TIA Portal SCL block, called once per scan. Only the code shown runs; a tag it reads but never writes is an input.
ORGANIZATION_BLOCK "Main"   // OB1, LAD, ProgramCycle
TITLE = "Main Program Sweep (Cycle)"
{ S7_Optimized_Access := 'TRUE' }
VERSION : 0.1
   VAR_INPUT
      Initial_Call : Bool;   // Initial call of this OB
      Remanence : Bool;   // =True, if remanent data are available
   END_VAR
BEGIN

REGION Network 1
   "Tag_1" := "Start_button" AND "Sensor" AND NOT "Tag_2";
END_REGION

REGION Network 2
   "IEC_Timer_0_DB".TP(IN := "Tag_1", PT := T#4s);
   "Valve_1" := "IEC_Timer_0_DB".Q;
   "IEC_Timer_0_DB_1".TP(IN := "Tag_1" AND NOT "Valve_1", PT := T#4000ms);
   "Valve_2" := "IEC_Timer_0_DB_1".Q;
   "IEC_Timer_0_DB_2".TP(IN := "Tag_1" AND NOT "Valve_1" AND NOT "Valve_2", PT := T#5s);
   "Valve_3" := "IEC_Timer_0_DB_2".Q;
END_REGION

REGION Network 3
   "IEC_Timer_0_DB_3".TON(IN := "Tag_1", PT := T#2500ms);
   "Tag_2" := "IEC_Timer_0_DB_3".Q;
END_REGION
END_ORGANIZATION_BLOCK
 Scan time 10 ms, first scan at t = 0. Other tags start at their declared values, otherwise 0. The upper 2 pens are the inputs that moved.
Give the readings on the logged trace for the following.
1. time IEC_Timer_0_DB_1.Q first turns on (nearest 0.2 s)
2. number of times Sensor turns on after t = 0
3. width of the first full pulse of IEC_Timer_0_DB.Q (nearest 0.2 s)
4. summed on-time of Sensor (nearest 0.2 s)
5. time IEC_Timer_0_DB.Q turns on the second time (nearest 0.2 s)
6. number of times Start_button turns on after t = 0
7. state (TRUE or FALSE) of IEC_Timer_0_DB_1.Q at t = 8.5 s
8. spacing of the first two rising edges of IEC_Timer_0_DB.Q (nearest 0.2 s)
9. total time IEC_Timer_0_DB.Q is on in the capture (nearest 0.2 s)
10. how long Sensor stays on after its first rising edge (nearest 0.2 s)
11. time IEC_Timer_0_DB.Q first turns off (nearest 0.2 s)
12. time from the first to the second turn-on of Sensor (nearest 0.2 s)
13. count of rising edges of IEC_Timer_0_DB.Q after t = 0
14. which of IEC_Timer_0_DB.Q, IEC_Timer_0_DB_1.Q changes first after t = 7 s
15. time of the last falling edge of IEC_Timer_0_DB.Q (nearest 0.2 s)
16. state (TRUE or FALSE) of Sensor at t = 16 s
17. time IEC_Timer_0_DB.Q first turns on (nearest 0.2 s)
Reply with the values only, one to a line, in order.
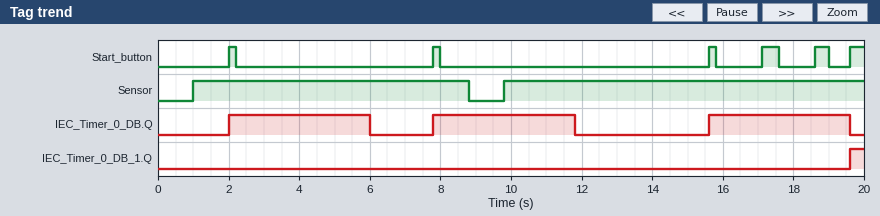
19.6 s
2
4.0 s
18.0 s
7.8 s
6
FALSE
5.8 s
12.0 s
7.8 s
6.0 s
8.8 s
3
IEC_Timer_0_DB.Q
19.6 s
TRUE
2.0 s
